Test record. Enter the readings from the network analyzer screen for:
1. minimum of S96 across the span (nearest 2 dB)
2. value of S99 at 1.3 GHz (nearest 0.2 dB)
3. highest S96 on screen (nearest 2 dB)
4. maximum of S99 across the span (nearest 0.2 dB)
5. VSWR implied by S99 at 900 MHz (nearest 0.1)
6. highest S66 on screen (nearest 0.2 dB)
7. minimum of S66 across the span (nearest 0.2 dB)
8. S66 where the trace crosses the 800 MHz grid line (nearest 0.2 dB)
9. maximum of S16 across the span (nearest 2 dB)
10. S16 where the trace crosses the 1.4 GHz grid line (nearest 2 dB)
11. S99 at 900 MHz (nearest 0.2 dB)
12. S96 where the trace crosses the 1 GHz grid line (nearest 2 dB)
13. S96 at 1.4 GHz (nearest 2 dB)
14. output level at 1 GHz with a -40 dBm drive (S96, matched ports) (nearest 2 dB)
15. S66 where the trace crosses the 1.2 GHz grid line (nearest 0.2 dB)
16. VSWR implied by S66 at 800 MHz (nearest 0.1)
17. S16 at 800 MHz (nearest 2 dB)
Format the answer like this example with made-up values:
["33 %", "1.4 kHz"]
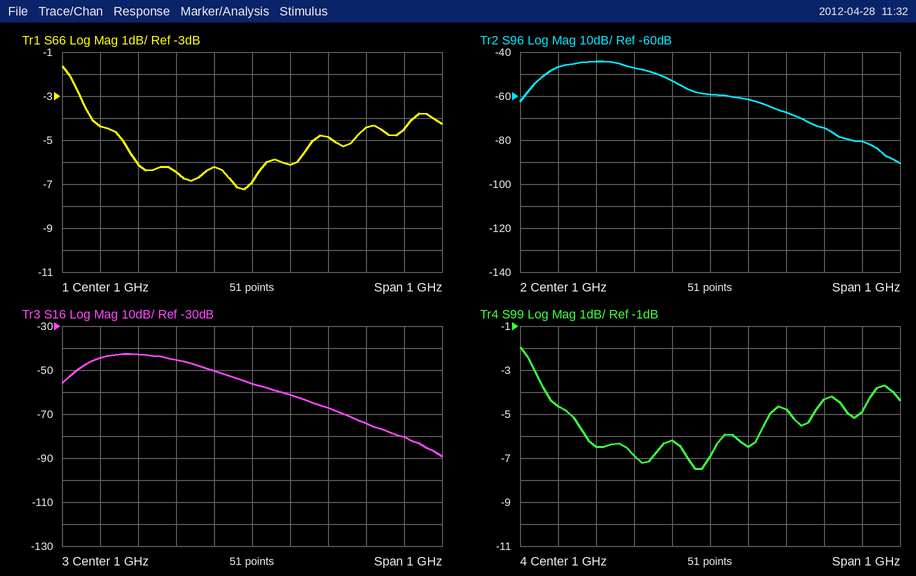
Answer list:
["-90 dB", "-4.4 dB", "-44 dB", "-2.0 dB", "2.9", "-1.6 dB", "-7.2 dB", "-6.4 dB", "-42 dB", "-80 dB", "-6.2 dB", "-60 dB", "-80 dB", "-100 dBm", "-4.8 dB", "2.8", "-46 dB"]
